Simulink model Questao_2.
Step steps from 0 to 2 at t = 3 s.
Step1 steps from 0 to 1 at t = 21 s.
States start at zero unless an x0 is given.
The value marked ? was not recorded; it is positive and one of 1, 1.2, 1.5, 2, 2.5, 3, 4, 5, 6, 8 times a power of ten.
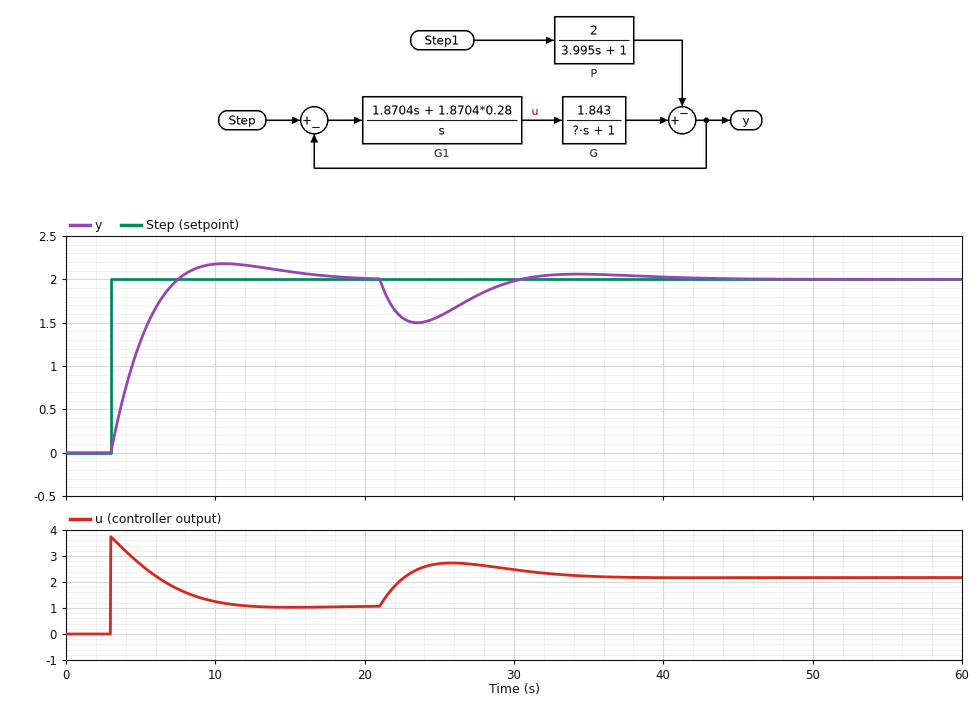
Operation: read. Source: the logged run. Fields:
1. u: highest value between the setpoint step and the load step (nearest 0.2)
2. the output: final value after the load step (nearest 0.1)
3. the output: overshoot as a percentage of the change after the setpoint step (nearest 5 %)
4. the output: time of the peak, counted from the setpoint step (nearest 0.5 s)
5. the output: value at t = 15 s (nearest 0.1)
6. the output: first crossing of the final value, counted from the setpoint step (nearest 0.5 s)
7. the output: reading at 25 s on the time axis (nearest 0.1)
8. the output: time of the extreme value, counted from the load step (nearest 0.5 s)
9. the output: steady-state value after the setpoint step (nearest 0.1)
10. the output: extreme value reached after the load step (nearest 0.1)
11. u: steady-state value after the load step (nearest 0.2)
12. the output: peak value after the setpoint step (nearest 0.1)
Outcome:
3.8
2.0
10 %
7.5 s
2.1
4.5 s
1.6
2.5 s
2.0
1.5
2.2
2.2
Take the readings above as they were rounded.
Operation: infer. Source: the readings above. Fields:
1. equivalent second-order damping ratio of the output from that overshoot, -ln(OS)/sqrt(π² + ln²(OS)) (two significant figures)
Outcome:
0.59
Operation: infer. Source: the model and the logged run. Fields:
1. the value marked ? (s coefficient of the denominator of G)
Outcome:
8
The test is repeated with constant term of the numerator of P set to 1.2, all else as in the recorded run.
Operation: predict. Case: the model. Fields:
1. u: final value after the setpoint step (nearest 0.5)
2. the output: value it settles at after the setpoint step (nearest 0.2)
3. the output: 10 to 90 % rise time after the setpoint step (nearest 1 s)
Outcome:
1.0
2.0
3 s
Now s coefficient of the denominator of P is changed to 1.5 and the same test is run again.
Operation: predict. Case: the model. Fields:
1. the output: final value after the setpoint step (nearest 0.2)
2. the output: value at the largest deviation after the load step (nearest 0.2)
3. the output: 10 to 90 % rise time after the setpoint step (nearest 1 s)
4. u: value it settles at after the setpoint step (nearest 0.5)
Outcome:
2.0
1.2
3 s
1.0
